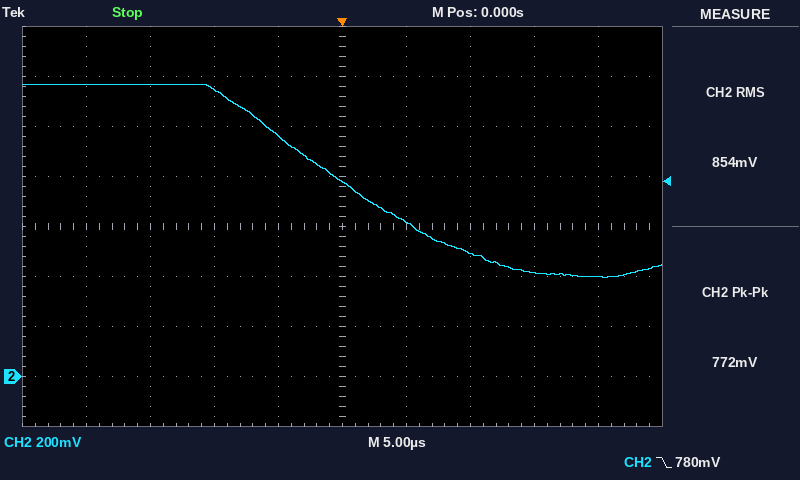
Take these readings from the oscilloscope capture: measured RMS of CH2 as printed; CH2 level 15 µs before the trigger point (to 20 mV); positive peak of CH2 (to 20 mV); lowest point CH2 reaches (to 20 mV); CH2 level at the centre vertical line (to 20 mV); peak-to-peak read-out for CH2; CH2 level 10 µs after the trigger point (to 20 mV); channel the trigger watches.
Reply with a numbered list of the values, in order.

1. 854 mV
2. 1.16 V
3. 1.16 V
4. 400 mV
5. 780 mV
6. 772 mV
7. 500 mV
8. CH2
